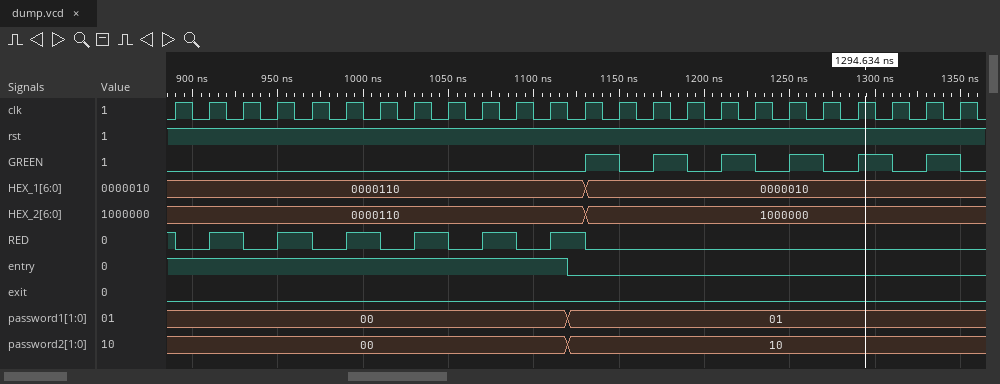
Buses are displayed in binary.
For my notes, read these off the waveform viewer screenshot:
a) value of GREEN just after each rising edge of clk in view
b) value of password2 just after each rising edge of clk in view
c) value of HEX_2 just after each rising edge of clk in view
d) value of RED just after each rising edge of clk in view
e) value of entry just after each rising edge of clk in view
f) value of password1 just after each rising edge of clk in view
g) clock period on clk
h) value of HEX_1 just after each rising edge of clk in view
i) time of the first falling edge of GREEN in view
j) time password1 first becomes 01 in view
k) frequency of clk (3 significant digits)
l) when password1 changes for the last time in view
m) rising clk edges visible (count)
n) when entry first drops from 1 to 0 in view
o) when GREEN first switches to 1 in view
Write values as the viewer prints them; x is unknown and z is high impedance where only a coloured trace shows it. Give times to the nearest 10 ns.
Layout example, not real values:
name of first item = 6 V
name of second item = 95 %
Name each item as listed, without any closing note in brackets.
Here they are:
value of GREEN just after each rising edge of clk in view = 0 0 0 0 0 0 0 0 0 0 0 0 1 0 1 0 1 0 1 0 1 0 1 0
value of password2 just after each rising edge of clk in view = 00, 00, 00, 00, 00, 00, 00, 00, 00, 00, 00, 00, 10, 10, 10, 10, 10, 10, 10, 10, 10, 10, 10, 10
value of HEX_2 just after each rising edge of clk in view = 0000110, 0000110, 0000110, 0000110, 0000110, 0000110, 0000110, 0000110, 0000110, 0000110, 0000110, 0000110, 1000000, 1000000, 1000000, 1000000, 1000000, 1000000, 1000000, 1000000, 1000000, 1000000, 1000000, 1000000
value of RED just after each rising edge of clk in view = 0 1 0 1 0 1 0 1 0 1 0 1 0 0 0 0 0 0 0 0 0 0 0 0
value of entry just after each rising edge of clk in view = 1 1 1 1 1 1 1 1 1 1 1 1 0 0 0 0 0 0 0 0 0 0 0 0
value of password1 just after each rising edge of clk in view = 00, 00, 00, 00, 00, 00, 00, 00, 00, 00, 00, 00, 01, 01, 01, 01, 01, 01, 01, 01, 01, 01, 01, 01
clock period on clk = 20 ns
value of HEX_1 just after each rising edge of clk in view = 0000110, 0000110, 0000110, 0000110, 0000110, 0000110, 0000110, 0000110, 0000110, 0000110, 0000110, 0000110, 0000010, 0000010, 0000010, 0000010, 0000010, 0000010, 0000010, 0000010, 0000010, 0000010, 0000010, 0000010
time of the first falling edge of GREEN in view = 1150 ns
time password1 first becomes 01 in view = 1120 ns
frequency of clk = 50.0 MHz
when password1 changes for the last time in view = 1120 ns
rising clk edges visible = 24
when entry first drops from 1 to 0 in view = 1120 ns
when GREEN first switches to 1 in view = 1130 ns
